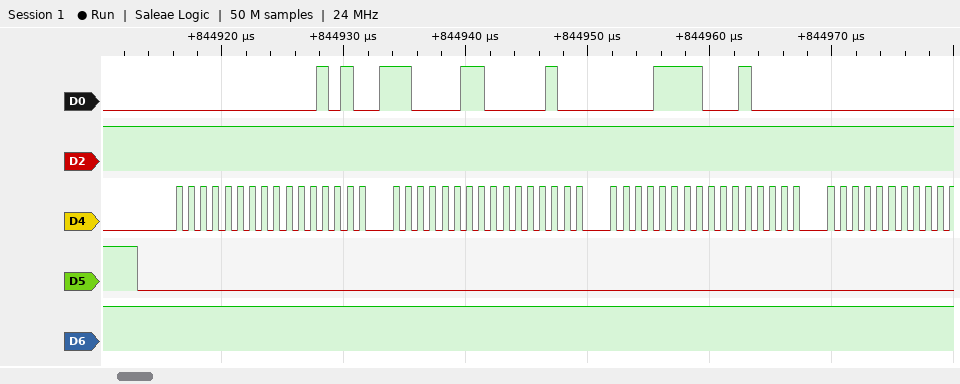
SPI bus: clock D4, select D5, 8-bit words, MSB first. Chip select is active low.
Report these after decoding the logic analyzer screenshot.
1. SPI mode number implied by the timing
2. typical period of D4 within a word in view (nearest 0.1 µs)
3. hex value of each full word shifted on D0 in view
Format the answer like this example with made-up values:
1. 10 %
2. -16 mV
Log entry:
1. 0
2. 1 µs
3. 00, 0A, C3, 04, 0F, 10, 00
